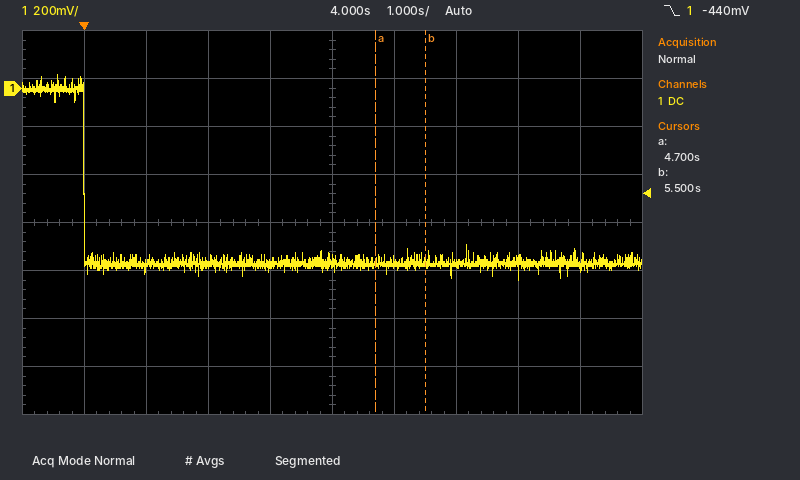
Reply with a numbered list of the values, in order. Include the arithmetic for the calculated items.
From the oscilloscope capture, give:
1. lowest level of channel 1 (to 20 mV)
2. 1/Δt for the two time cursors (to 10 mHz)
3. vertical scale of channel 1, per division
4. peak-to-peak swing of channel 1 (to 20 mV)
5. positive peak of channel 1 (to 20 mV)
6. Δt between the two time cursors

1. -800 mV
2. 1 / 800 ms ≈ 1.25 Hz
3. 200 mV
4. 60 mV − (-800 mV) = 860 mV
5. 60 mV
6. 5.5 s − (4.7 s) = 800 ms
